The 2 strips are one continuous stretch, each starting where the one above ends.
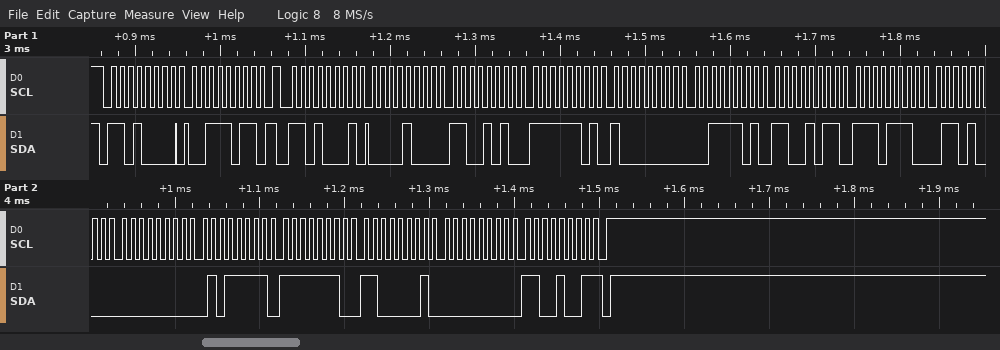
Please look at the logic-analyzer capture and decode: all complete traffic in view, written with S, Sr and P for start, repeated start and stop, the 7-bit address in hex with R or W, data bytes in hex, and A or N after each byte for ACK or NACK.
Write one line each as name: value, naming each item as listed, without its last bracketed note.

all complete traffic in view, written with S, Sr and P for start, repeated start and stop, the 7-bit address in hex with R or W, data bytes in hex, and A or N after each byte for ACK or NACK: S 68W A 3B A Sr 68R A 08 A CA A FD A 80 A 3D A CB A EE A 68 A 00 A 5F A FE A C1 A 00 A C9 N P
